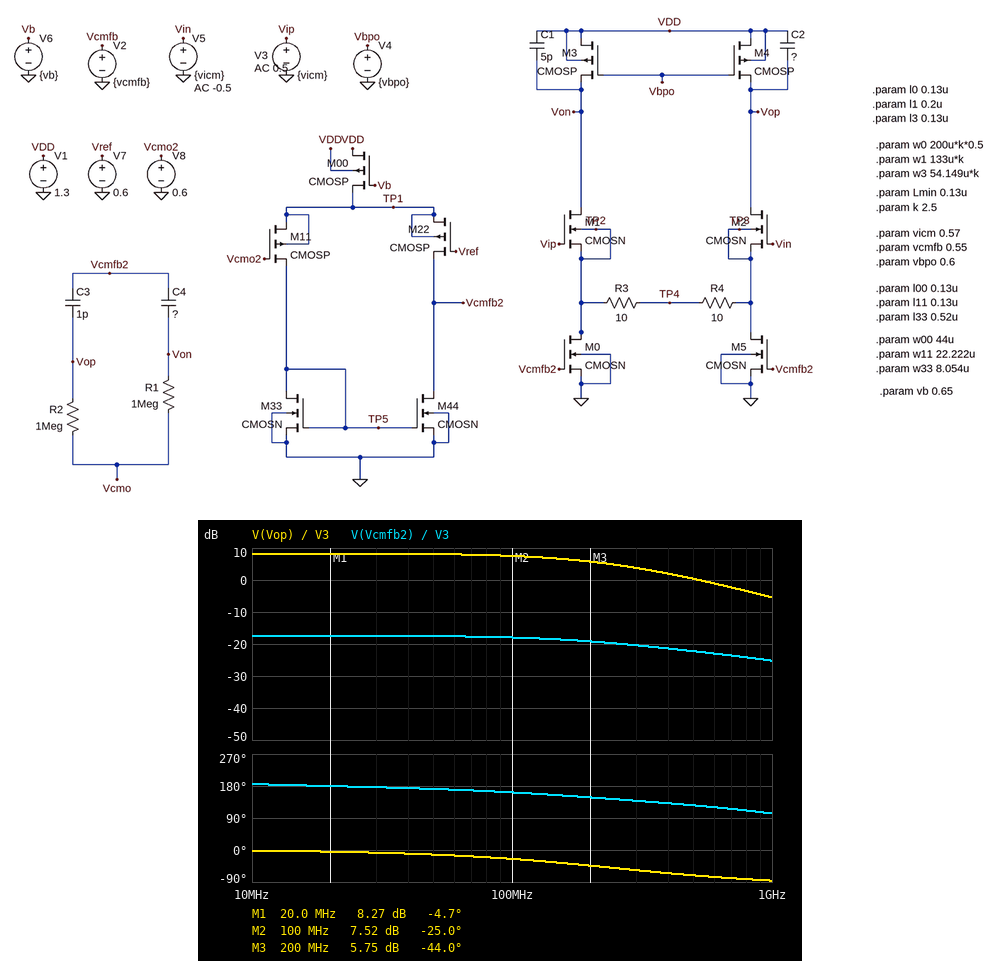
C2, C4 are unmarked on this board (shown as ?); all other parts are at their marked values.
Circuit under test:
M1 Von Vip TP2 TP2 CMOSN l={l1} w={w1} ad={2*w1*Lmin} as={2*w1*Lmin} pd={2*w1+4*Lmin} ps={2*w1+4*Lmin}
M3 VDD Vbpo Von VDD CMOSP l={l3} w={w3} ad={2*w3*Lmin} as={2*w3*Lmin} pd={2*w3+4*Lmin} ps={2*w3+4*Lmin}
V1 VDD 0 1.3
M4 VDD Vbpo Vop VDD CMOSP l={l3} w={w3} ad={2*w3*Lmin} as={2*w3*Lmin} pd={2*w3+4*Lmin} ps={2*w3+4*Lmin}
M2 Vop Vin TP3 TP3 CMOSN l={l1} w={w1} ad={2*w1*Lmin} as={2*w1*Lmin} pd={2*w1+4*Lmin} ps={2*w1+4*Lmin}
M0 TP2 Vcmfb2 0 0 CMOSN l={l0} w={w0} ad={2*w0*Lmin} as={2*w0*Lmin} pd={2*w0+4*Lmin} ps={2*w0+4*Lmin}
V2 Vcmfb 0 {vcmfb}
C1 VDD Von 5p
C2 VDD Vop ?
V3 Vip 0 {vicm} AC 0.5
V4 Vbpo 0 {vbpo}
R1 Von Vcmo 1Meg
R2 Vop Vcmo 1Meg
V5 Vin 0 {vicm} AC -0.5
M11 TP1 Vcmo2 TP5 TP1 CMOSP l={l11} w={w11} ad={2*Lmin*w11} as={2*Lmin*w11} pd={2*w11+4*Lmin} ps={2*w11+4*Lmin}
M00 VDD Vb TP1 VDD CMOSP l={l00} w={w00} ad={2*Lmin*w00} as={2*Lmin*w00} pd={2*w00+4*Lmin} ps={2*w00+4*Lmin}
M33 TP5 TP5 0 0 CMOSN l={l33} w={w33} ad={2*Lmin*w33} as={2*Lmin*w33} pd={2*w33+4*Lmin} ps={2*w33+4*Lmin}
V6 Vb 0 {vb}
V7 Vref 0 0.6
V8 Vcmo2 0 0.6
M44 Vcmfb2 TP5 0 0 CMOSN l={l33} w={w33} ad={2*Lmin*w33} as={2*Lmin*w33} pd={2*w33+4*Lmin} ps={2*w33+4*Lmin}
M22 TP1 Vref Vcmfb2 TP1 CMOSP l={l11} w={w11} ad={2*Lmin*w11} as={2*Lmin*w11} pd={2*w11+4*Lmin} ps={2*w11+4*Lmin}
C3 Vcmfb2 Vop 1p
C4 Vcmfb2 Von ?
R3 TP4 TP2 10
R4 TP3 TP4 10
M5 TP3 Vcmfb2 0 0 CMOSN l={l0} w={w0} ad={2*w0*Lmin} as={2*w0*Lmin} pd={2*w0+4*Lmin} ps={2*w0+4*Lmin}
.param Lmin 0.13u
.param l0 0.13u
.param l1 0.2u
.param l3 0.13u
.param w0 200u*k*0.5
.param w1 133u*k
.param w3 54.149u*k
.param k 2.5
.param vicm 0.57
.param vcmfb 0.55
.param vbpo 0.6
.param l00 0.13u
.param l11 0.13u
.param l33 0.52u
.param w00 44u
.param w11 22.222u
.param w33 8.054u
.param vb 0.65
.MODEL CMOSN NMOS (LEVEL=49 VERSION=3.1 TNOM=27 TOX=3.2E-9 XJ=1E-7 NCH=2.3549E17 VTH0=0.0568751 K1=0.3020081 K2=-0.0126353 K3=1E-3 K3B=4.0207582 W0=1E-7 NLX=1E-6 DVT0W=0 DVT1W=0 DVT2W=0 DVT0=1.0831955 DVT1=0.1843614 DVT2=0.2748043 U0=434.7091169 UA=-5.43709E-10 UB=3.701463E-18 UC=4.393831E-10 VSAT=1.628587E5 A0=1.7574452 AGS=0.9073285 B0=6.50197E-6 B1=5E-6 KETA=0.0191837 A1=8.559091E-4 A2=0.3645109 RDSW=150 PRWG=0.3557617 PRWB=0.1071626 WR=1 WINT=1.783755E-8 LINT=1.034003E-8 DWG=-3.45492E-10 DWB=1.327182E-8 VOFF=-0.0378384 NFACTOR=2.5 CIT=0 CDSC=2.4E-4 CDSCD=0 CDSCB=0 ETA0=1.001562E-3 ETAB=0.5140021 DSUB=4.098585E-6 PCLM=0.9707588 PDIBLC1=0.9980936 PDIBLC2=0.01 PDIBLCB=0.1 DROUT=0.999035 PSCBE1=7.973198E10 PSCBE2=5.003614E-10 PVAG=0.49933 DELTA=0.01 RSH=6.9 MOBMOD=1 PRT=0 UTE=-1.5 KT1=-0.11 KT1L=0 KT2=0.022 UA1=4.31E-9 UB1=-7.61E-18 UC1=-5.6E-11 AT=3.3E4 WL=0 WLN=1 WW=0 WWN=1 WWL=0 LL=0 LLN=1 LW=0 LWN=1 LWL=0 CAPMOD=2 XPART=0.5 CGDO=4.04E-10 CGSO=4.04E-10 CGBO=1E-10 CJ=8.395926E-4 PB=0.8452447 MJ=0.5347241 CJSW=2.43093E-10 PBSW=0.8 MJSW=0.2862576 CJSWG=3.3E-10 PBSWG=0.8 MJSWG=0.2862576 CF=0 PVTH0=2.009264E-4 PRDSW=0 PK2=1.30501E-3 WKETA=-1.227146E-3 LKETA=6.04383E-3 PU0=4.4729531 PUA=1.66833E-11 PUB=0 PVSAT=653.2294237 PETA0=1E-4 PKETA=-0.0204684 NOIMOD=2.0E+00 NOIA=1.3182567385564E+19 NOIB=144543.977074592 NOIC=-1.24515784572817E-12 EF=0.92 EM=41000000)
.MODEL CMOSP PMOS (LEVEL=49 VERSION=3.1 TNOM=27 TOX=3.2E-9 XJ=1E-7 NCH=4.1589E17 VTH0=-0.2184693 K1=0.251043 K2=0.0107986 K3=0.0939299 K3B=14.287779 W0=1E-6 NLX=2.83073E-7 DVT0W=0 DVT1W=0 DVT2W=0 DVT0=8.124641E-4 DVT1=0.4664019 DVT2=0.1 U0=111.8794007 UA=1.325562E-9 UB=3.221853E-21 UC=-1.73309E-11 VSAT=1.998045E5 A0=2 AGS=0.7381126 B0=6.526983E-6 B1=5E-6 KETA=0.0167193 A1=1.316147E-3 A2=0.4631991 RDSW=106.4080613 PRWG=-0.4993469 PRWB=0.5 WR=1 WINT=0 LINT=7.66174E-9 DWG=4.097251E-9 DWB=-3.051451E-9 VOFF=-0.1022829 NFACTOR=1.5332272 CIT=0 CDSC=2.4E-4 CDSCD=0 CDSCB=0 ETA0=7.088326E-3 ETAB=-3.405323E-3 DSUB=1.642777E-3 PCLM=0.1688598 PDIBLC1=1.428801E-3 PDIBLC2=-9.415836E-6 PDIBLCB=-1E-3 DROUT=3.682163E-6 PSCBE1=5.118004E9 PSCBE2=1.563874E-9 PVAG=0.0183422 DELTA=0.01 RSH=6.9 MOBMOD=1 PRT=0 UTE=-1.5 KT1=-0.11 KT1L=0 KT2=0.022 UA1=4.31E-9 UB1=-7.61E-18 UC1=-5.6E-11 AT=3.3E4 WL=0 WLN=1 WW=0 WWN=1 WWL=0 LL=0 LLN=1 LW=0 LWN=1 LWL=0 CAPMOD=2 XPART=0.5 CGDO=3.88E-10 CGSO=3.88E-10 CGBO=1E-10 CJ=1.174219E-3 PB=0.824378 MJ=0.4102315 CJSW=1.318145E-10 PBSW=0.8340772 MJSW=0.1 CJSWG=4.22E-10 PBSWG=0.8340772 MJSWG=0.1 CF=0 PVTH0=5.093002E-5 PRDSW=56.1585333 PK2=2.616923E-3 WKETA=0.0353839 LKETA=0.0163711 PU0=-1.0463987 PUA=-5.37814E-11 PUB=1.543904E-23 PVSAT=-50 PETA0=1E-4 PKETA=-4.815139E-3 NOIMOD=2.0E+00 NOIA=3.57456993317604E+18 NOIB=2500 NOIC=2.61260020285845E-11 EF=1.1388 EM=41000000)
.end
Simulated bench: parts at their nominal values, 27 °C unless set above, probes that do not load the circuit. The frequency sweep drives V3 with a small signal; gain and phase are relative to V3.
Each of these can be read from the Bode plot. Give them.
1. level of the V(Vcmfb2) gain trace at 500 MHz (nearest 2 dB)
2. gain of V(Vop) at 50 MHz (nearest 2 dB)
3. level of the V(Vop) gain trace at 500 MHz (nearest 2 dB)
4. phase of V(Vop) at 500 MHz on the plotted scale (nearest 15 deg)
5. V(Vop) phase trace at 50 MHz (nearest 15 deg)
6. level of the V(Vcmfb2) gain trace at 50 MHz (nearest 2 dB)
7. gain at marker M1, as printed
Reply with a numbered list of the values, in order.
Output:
1. -22 dB
2. 8 dB
3. 0 dB
4. -75 deg
5. -15 deg
6. -18 dB
7. 8.27 dB
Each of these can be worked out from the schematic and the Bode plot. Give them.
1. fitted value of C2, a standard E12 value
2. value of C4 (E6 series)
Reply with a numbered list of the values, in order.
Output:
1. 3.9 pF
2. 1.5 pF
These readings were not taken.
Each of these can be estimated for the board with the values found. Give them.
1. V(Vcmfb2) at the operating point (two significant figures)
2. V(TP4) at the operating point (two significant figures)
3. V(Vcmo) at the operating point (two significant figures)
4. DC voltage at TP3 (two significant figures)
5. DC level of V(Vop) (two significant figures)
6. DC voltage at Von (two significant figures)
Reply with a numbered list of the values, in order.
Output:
1. 550 mV
2. 130 mV
3. 1.1 V
4. 130 mV
5. 1.1 V
6. 1.1 V
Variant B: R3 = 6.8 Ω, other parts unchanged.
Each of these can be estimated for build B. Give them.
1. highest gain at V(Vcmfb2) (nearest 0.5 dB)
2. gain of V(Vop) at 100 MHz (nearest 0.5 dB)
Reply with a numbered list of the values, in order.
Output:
1. -17.0 dB
2. 8.0 dB
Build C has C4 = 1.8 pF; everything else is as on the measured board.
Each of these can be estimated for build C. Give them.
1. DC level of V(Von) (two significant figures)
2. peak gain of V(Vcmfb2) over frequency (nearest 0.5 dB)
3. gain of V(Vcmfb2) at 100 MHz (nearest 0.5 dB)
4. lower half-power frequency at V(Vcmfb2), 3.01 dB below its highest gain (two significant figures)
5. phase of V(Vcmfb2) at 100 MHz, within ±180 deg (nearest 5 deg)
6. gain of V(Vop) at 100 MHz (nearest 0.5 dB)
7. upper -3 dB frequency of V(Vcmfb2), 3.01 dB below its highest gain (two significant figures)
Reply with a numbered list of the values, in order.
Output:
1. 1.1 V
2. -15.0 dB
3. -15.5 dB
4. 1.2 MHz
5. 165 deg
6. 8.0 dB
7. 340 MHz
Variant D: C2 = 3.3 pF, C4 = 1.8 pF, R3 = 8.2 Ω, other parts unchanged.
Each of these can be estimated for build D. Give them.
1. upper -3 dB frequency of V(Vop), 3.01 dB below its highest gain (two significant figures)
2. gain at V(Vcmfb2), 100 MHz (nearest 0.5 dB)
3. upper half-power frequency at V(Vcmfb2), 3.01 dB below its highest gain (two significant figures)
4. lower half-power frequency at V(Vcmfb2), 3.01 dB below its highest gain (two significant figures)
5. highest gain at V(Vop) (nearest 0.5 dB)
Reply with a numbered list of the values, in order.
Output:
1. 240 MHz
2. -15.5 dB
3. 280 MHz
4. 1.2 MHz
5. 9.0 dB
